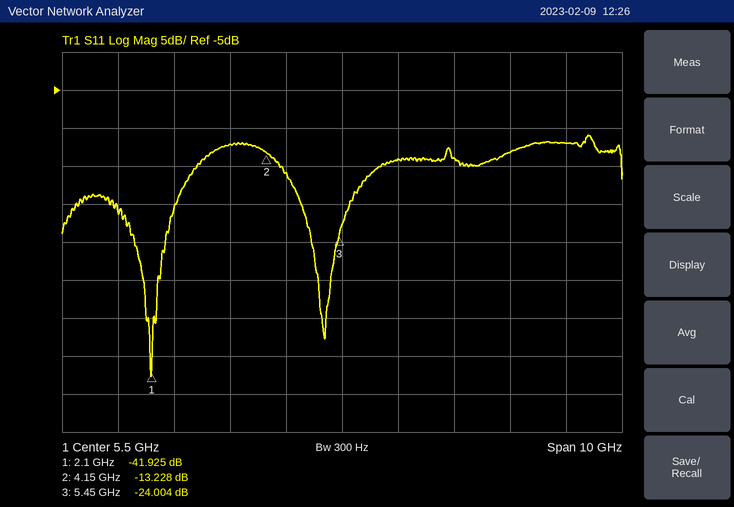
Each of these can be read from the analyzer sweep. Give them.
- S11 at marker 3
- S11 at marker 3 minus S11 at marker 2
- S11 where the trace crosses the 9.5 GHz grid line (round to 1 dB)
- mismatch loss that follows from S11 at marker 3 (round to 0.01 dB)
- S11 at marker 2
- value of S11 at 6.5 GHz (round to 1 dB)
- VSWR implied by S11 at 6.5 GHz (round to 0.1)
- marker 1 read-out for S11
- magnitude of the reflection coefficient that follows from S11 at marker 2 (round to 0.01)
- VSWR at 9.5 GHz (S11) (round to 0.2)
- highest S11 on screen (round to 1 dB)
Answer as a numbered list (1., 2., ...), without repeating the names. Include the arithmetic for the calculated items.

1. -24.004 dB
2. -24.004 − (-13.228) = -10.776 dB
3. -12 dB
4. −10 log10(1 − 10^(-24.004/10)) ≈ 0.02 dB
5. -13.228 dB
6. -14 dB
7. |Γ| = 10^(-14/20) = 0.1995; VSWR = (1 + 0.1995)/(1 − 0.1995) ≈ 1.5
8. -41.925 dB
9. 10^(-13.228/20) ≈ 0.22
10. |Γ| = 10^(-12/20) = 0.2512; VSWR = (1 + 0.2512)/(1 − 0.2512) ≈ 1.67, so 1.6 to the nearest 0.2
11. -11 dB
